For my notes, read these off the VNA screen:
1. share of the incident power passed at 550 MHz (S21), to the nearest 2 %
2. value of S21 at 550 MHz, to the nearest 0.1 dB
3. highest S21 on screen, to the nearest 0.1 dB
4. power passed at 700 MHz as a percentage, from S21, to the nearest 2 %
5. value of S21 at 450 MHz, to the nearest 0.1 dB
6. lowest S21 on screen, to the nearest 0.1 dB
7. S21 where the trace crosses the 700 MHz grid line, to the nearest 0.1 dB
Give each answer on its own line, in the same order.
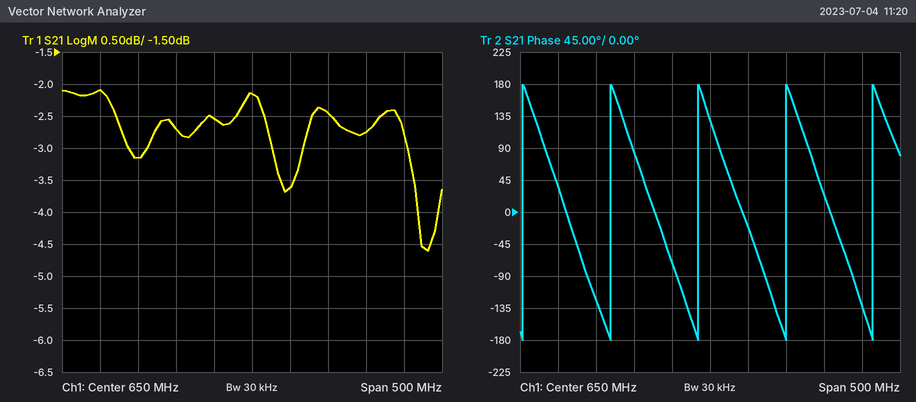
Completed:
54 %
-2.7 dB
-2.1 dB
44 %
-2.1 dB
-4.6 dB
-3.6 dB
